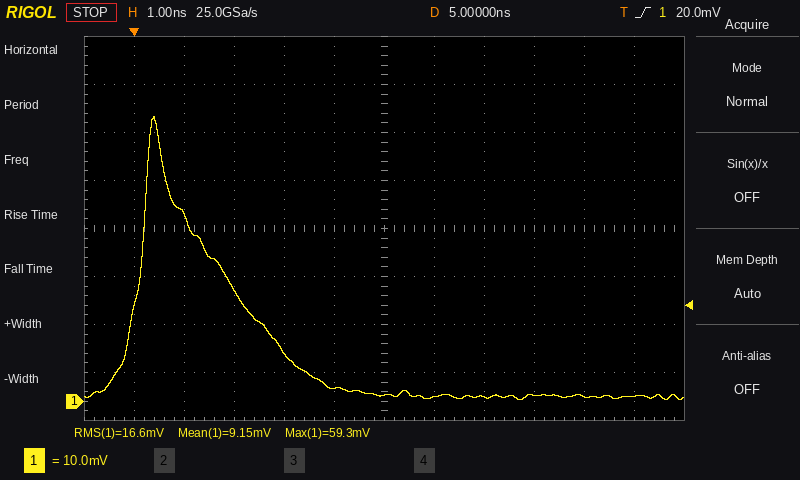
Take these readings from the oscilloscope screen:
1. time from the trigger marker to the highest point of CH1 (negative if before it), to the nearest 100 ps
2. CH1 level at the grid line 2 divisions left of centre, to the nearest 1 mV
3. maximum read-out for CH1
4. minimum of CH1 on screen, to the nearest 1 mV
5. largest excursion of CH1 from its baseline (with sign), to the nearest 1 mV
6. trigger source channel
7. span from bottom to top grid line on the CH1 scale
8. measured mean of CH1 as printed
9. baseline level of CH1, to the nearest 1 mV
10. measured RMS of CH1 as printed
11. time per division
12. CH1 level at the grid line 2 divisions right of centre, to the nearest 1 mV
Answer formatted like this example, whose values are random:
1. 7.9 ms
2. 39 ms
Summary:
1. +400 ps
2. 10 mV
3. 59.3 mV
4. 0 mV
5. +58 mV
6. CH1
7. 80 mV
8. 9.15 mV
9. 1 mV
10. 16.6 mV
11. 1 ns
12. 1 mV
